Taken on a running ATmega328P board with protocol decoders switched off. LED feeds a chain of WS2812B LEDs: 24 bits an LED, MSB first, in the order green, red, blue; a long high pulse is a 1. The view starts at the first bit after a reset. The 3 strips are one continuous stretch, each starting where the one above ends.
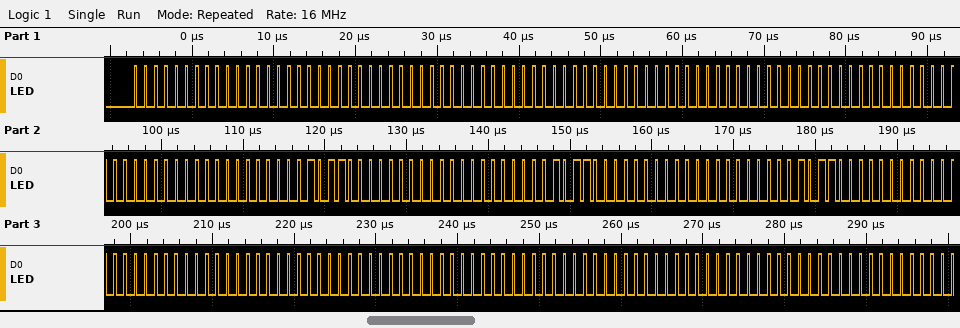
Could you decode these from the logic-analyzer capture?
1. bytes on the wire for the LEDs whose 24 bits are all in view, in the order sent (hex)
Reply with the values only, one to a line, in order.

00 00 00 00 00 00 00 00 00 00 00 00 0B 00 00 0B 00 00 0B 00 00 00 00 00 00 00 00 00 00 00
